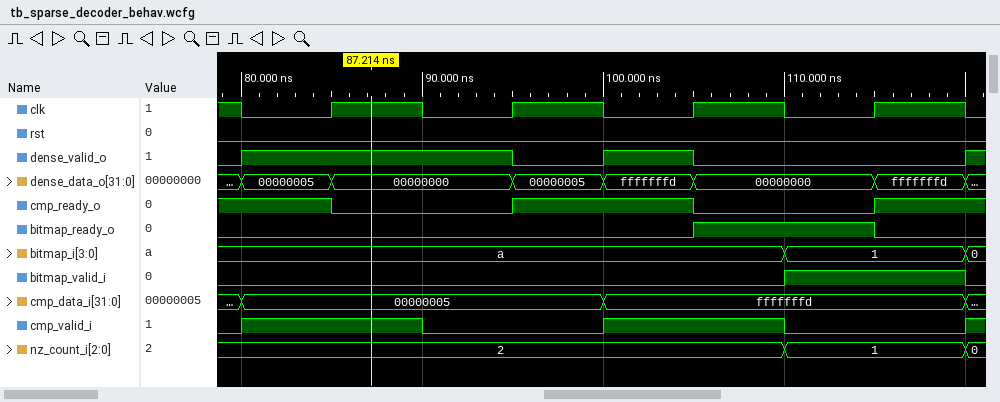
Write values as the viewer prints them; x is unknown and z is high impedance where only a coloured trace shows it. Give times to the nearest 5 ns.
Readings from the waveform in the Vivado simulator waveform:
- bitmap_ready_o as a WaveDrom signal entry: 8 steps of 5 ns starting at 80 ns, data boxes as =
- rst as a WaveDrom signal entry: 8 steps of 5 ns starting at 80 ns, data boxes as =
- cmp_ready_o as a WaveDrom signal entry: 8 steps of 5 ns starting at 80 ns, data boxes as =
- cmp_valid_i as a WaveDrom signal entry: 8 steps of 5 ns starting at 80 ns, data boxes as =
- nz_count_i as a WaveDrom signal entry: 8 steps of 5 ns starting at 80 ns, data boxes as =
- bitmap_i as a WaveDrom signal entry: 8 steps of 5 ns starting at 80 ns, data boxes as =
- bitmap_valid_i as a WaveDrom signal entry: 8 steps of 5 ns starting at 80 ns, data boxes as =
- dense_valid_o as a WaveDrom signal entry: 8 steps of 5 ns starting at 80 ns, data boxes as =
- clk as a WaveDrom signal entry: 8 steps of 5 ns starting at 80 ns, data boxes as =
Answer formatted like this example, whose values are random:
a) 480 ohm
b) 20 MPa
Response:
a) {name: 'bitmap_ready_o', wave: '0....1.0'}
b) {name: 'rst', wave: '0.......'}
c) {name: 'cmp_ready_o', wave: '10.1.0.1'}
d) {name: 'cmp_valid_i', wave: '1.0.1.0.'}
e) {name: 'nz_count_i', wave: '=.....=.', data: '2 1'}
f) {name: 'bitmap_i', wave: '=.....=.', data: 'a 1'}
g) {name: 'bitmap_valid_i', wave: '0.....1.'}
h) {name: 'dense_valid_o', wave: '1..010..'}
i) {name: 'clk', wave: '01010101'}
